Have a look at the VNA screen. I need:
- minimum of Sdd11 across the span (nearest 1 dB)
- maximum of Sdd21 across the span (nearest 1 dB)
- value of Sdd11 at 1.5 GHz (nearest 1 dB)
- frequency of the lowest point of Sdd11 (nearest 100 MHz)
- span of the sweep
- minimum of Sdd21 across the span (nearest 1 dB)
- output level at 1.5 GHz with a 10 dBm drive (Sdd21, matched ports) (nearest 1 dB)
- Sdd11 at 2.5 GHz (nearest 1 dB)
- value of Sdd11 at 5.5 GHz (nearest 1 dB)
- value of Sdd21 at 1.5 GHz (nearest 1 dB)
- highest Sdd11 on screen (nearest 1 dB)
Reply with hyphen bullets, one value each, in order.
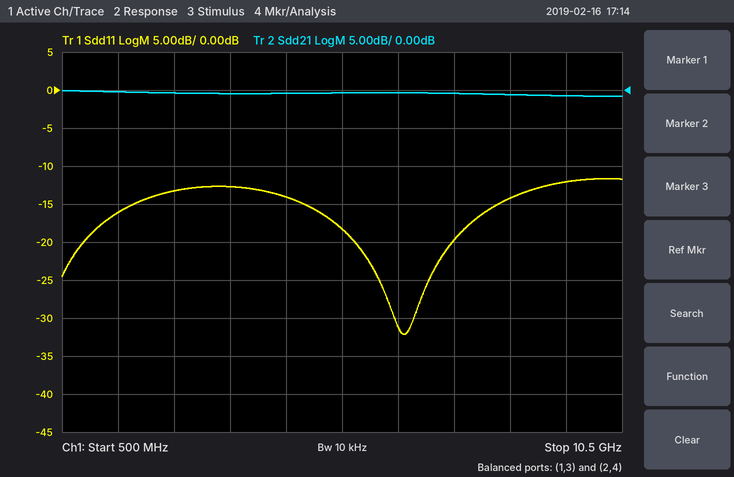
- -32 dB
- 0 dB
- -16 dB
- 6.6 GHz
- 10 GHz
- -1 dB
- 10 dBm
- -13 dB
- -18 dB
- 0 dB
- -12 dB
